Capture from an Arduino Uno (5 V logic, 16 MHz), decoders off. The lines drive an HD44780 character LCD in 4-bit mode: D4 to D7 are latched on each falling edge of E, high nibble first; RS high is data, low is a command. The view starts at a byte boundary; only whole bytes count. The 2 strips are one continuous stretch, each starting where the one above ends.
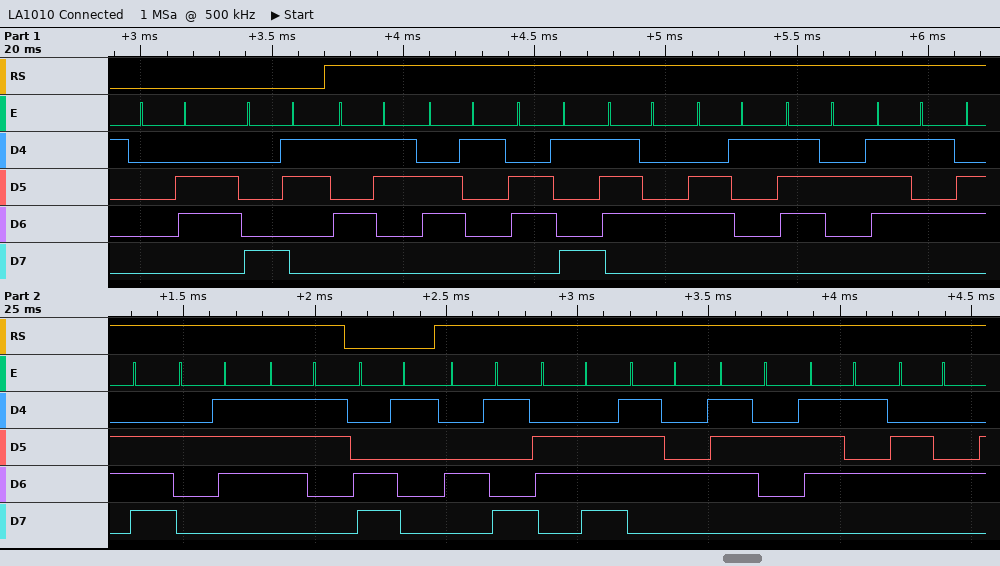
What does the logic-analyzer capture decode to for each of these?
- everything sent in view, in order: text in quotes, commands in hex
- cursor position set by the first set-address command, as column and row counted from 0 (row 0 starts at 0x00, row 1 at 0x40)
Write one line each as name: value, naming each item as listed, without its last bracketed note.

everything sent in view, in order: text in quotes, commands in hex: 0x06 0x83 "Saitarun's" 0xC1 "Intrud"
cursor position set by the first set-address command, as column and row counted from 0: column 3, row 0
